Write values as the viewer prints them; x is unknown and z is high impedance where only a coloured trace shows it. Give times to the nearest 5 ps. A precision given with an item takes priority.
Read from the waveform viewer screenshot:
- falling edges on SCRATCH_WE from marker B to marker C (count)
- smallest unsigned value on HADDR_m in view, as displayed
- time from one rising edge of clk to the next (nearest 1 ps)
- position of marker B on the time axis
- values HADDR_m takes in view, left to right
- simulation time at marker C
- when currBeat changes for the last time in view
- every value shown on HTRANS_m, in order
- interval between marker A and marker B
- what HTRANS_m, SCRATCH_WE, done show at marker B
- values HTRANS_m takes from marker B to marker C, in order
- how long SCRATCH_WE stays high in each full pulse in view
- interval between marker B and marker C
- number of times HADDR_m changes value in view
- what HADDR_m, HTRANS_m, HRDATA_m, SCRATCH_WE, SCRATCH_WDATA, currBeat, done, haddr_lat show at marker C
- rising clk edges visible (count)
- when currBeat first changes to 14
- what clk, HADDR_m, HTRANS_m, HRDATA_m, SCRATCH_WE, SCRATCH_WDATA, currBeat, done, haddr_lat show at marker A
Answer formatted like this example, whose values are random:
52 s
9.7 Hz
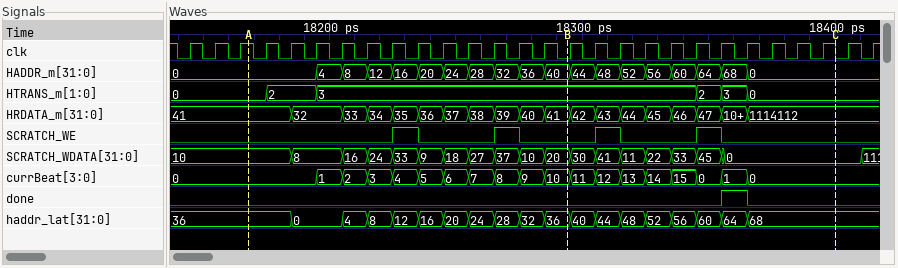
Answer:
2
0
10 ps
18295 ps
0, 4, 8, 12, 16, 20, 24, 28, 32, 36, 40, 44, 48, 52, 56, 60, 64, 68, 0
18400 ps
18365 ps
0, 2, 3, 2, 3, 0
125 ps
HTRANS_m=3, SCRATCH_WE=0, done=0
3, 2, 3, 0
10 ps, 10 ps, 10 ps, 10 ps
105 ps
18
HADDR_m=0, HTRANS_m=0, HRDATA_m=1114112, SCRATCH_WE=0, SCRATCH_WDATA=0, currBeat=0, done=0, haddr_lat=68
28
18325 ps
clk=1, HADDR_m=0, HTRANS_m=0, HRDATA_m=41, SCRATCH_WE=0, SCRATCH_WDATA=10, currBeat=0, done=0, haddr_lat=36
